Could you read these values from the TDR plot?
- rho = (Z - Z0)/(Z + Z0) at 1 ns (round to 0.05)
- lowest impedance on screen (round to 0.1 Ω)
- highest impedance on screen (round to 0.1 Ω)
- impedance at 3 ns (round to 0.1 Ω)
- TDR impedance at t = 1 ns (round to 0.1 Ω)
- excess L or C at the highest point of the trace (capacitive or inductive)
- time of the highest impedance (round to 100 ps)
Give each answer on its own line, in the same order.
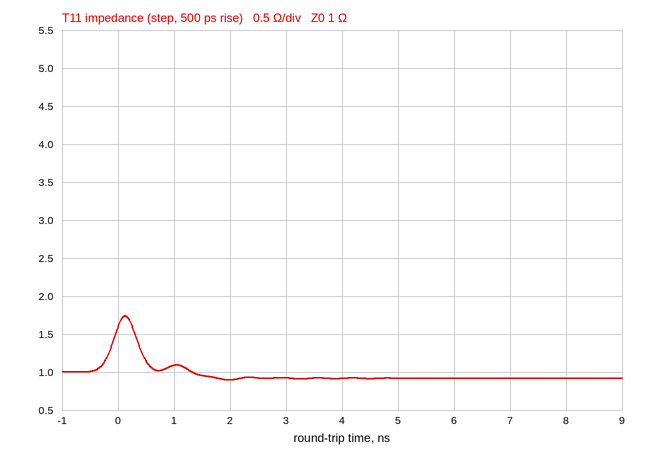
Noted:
+0.05
0.9 Ω
1.7 Ω
0.9 Ω
1.1 Ω
inductive
100 ps
